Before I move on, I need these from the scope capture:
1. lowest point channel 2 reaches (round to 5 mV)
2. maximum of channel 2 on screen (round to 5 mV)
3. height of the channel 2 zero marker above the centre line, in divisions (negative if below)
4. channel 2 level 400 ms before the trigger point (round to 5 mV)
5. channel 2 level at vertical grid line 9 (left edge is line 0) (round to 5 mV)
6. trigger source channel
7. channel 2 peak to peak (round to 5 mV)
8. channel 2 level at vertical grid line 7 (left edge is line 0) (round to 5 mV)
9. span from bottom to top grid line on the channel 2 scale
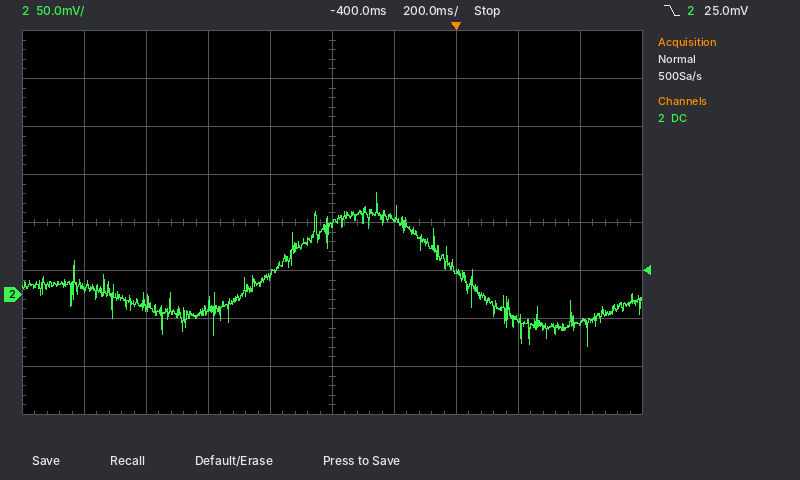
-55 mV
105 mV
-1.5 div
75 mV
-30 mV
channel 2
160 mV
25 mV
400 mV
